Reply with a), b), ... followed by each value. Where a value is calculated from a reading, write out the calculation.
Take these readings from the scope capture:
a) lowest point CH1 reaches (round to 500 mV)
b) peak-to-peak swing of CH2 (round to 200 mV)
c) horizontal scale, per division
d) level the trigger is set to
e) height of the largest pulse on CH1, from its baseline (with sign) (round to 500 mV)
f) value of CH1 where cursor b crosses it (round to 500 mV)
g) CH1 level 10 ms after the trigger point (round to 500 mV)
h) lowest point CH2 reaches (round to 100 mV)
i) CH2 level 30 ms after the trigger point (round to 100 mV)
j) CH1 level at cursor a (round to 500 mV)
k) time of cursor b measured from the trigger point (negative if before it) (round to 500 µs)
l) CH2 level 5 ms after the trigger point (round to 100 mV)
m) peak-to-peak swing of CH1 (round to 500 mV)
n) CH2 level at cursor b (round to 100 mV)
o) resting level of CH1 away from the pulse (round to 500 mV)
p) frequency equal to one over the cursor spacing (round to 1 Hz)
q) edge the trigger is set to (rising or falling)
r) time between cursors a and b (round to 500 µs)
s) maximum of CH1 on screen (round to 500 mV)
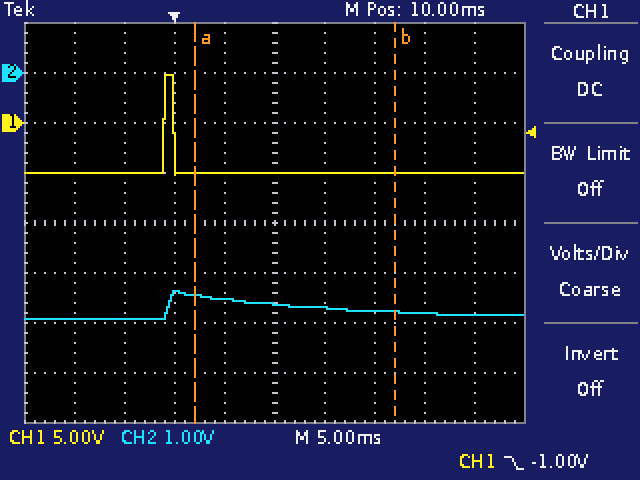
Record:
a) -5.0 V
b) 600 mV
c) 5 ms
d) -1.00 V
e) 5.0 V − (-5.0 V) = +10.0 V
f) -5.0 V
g) -5.0 V
h) -4.9 V
i) -4.8 V
j) -5.0 V
k) +22.0 ms
l) -4.5 V
m) 5.0 V − (-5.0 V) = 10.0 V
n) -4.8 V
o) -5.0 V
p) 1 / 20.0 ms ≈ 50 Hz
q) falling
r) 20.0 ms
s) 5.0 V
